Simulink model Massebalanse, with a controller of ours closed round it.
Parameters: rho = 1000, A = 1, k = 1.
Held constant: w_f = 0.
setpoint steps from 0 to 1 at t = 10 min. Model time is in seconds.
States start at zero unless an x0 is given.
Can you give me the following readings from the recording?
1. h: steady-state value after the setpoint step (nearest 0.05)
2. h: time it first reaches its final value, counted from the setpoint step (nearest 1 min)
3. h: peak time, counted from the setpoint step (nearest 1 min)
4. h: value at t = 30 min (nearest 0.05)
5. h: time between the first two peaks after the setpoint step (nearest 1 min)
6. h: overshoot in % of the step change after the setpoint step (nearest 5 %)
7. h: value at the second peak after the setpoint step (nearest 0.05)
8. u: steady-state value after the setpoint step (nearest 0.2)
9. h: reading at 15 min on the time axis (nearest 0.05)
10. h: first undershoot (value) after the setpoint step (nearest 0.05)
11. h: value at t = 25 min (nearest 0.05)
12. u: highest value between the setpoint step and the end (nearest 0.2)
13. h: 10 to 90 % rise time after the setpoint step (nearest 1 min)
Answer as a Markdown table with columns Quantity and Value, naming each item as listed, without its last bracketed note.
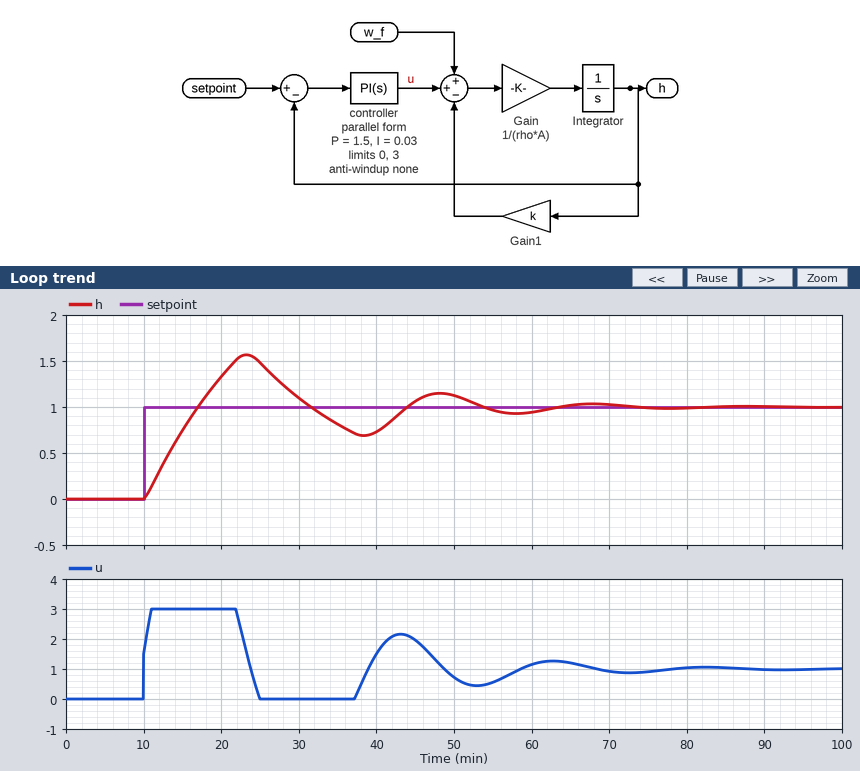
| Quantity | Value |
|---|---|
| h: steady-state value after the setpoint step | 1.00 |
| h: time it first reaches its final value, counted from the setpoint step | 7 min |
| h: peak time, counted from the setpoint step | 13 min |
| h: value at t = 30 min | 1.10 |
| h: time between the first two peaks after the setpoint step | 25 min |
| h: overshoot in % of the step change after the setpoint step | 55 % |
| h: value at the second peak after the setpoint step | 1.15 |
| u: steady-state value after the setpoint step | 1.0 |
| h: reading at 15 min on the time axis | 0.75 |
| h: first undershoot (value) after the setpoint step | 0.70 |
| h: value at t = 25 min | 1.50 |
| u: highest value between the setpoint step and the end | 3.0 |
| h: 10 to 90 % rise time after the setpoint step | 5 min |
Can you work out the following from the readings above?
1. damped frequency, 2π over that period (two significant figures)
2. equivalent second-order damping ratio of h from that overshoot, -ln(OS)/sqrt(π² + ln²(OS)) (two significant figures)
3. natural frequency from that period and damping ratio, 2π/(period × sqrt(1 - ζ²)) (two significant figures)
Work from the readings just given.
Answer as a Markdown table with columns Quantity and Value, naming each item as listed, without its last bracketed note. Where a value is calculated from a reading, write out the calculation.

| Quantity | Value |
|---|---|
| damped frequency, 2π over that period | 2π / 25 = 0.25 rad/min |
| equivalent second-order damping ratio of h from that overshoot, -ln(OS)/sqrt(π² + ln²(OS)) | ln(0.55) = -0.598; 0.598 / sqrt(9.870 + 0.357) = 0.19 |
| natural frequency from that period and damping ratio, 2π/(period × sqrt(1 - ζ²)) | 2π / (25 × sqrt(1 - 0.19²)) = 0.26 rad/min |
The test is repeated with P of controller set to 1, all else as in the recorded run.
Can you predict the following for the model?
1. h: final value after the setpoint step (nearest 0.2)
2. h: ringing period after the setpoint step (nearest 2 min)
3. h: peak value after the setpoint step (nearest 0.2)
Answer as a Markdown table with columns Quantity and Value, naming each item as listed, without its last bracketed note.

| Quantity | Value |
|---|---|
| h: final value after the setpoint step | 1.0 |
| h: ringing period after the setpoint step | 26 min |
| h: peak value after the setpoint step | 1.6 |
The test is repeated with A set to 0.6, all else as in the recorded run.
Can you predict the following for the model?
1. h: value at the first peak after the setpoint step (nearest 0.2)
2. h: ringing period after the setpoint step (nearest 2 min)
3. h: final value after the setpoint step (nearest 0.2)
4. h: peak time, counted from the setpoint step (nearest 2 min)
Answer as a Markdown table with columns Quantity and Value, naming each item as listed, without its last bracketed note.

| Quantity | Value |
|---|---|
| h: value at the first peak after the setpoint step | 1.4 |
| h: ringing period after the setpoint step | 16 min |
| h: final value after the setpoint step | 1.0 |
| h: peak time, counted from the setpoint step | 8 min |
